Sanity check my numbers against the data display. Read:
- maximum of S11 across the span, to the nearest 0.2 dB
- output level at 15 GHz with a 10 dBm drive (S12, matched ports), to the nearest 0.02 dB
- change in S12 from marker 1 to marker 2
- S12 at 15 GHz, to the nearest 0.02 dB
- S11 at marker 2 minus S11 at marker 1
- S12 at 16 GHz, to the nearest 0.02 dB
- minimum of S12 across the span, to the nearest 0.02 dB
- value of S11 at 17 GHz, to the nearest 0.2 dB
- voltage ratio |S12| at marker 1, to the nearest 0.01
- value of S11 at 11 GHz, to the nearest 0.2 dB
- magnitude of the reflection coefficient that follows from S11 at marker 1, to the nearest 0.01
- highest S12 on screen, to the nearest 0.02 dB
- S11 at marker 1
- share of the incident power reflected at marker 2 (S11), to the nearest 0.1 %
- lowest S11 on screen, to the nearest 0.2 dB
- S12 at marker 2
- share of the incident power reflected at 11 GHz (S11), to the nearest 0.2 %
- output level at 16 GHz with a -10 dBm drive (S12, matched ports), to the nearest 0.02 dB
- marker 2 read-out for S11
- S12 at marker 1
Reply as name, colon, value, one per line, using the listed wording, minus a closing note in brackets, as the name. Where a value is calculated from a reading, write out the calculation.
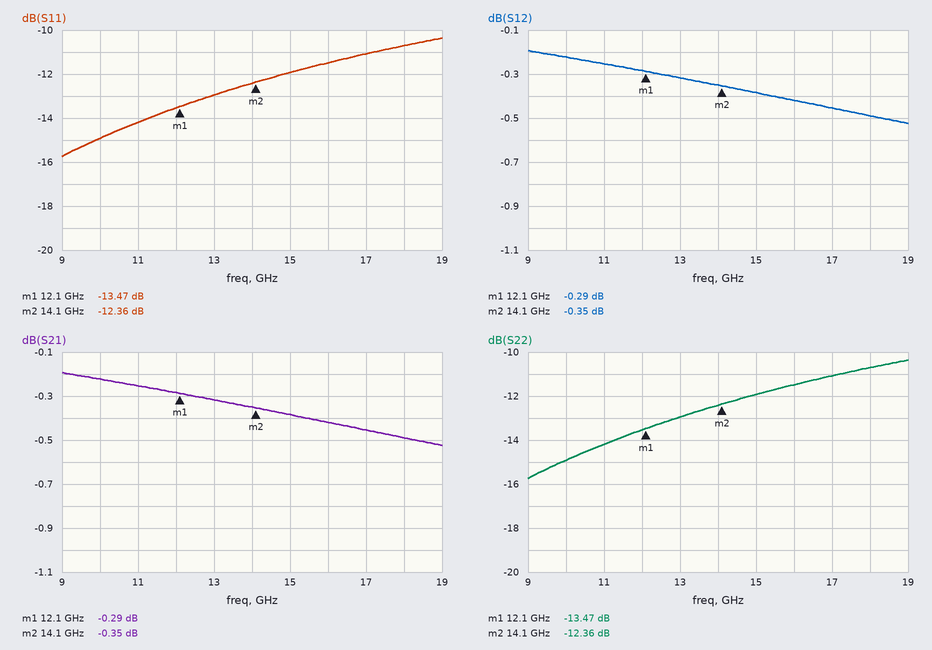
maximum of S11 across the span, to the nearest 0.2 dB: -10.4 dB
output level at 15 GHz with a 10 dBm drive (S12, matched ports), to the nearest 0.02 dB: 10 dBm + (-0.38 dB) = 9.62 dBm
change in S12 from marker 1 to marker 2: -0.35 − (-0.29) = -0.06 dB
S12 at 15 GHz, to the nearest 0.02 dB: -0.38 dB
S11 at marker 2 minus S11 at marker 1: -12.36 − (-13.47) = 1.11 dB
S12 at 16 GHz, to the nearest 0.02 dB: -0.42 dB
minimum of S12 across the span, to the nearest 0.02 dB: -0.52 dB
value of S11 at 17 GHz, to the nearest 0.2 dB: -11.0 dB
voltage ratio |S12| at marker 1, to the nearest 0.01: 10^(-0.29/20) ≈ 0.97
value of S11 at 11 GHz, to the nearest 0.2 dB: -14.2 dB
magnitude of the reflection coefficient that follows from S11 at marker 1, to the nearest 0.01: 10^(-13.47/20) ≈ 0.21
highest S12 on screen, to the nearest 0.02 dB: -0.20 dB
S11 at marker 1: -13.47 dB
share of the incident power reflected at marker 2 (S11), to the nearest 0.1 %: 10^(-12.36/10) ≈ 5.8 %
lowest S11 on screen, to the nearest 0.2 dB: -15.8 dB
S12 at marker 2: -0.35 dB
share of the incident power reflected at 11 GHz (S11), to the nearest 0.2 %: 10^(-14.2/10) ≈ 3.8 %
output level at 16 GHz with a -10 dBm drive (S12, matched ports), to the nearest 0.02 dB: -10 dBm + (-0.42 dB) = -10.42 dBm
marker 2 read-out for S11: -12.36 dB
S12 at marker 1: -0.29 dB
